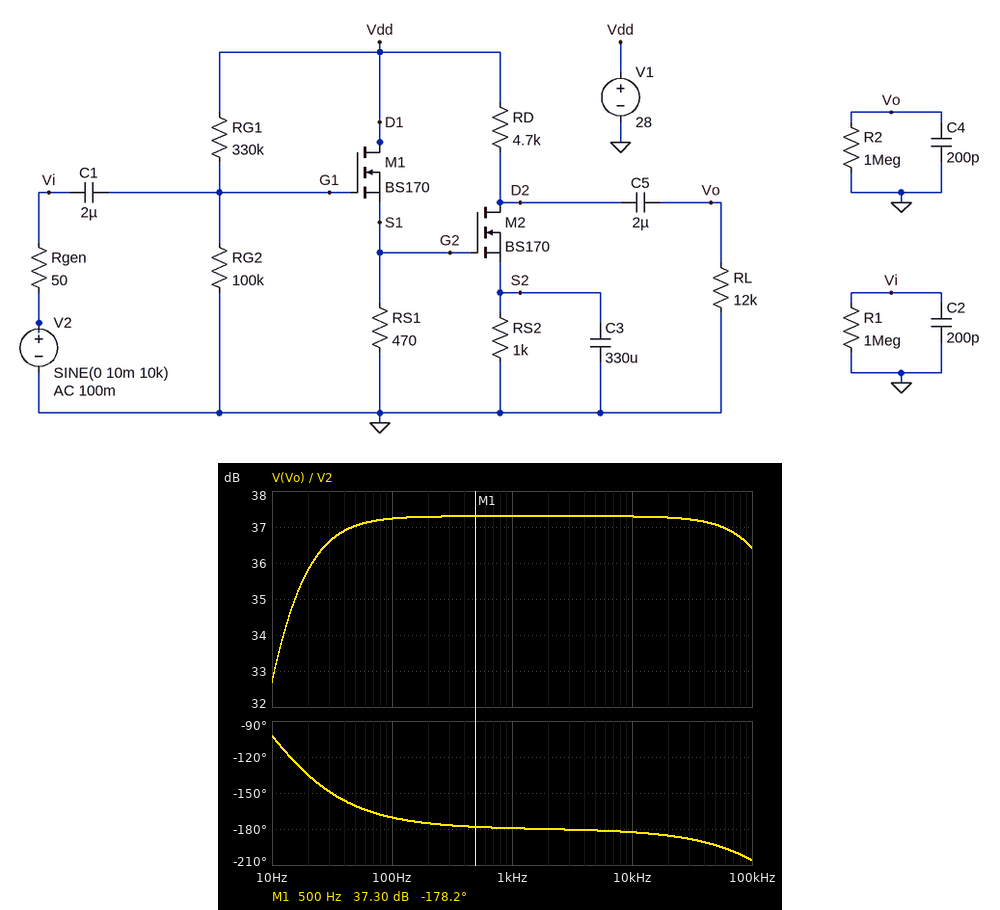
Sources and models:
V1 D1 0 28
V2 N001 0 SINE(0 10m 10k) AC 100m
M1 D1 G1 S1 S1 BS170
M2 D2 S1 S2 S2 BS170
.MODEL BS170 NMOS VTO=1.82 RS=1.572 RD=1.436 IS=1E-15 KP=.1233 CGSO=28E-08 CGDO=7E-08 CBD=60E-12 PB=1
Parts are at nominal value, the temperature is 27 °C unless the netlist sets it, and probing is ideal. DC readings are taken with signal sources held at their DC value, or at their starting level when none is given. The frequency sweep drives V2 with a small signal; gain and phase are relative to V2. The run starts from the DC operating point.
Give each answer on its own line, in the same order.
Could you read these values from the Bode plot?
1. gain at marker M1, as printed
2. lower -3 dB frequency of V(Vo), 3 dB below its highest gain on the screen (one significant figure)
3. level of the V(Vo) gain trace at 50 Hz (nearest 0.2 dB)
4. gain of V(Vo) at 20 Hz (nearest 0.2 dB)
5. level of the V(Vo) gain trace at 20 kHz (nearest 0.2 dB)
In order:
37.30 dB
10 Hz
37.0 dB
35.8 dB
37.2 dB
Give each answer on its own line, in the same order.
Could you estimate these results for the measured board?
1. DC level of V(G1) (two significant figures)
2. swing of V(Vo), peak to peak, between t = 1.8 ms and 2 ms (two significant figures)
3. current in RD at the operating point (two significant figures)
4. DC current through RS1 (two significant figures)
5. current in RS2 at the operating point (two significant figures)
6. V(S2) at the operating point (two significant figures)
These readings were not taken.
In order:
6.5 V
1.5 V
2.3 mA
9.1 mA
2.3 mA
2.3 V
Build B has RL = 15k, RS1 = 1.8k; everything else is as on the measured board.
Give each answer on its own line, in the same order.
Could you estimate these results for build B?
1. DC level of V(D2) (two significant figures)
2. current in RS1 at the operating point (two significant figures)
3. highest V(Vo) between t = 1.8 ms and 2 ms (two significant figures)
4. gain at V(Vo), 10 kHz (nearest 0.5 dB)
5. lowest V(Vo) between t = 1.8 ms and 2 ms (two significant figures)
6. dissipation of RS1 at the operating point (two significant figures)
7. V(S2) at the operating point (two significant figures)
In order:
16 V
2.5 mA
810 mV
38.5 dB
-840 mV
11 mW
2.5 V
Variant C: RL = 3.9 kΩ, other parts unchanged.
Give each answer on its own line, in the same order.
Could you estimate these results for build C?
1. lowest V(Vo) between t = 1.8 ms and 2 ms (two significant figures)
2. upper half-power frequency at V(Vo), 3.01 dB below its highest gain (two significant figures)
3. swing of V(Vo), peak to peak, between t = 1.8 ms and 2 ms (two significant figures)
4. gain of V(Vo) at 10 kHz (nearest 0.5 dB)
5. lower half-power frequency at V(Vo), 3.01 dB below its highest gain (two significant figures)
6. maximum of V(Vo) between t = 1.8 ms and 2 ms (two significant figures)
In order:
-470 mV
330 kHz
930 mV
33.5 dB
16 Hz
450 mV
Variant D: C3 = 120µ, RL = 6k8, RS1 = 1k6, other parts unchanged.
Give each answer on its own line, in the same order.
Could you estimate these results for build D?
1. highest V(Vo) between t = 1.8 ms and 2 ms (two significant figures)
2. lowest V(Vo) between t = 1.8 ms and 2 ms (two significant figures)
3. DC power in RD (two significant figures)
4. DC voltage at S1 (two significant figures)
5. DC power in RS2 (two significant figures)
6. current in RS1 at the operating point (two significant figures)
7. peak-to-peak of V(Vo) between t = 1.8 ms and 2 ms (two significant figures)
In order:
630 mV
-650 mV
28 mW
4.5 V
6.0 mW
2.8 mA
1.3 V
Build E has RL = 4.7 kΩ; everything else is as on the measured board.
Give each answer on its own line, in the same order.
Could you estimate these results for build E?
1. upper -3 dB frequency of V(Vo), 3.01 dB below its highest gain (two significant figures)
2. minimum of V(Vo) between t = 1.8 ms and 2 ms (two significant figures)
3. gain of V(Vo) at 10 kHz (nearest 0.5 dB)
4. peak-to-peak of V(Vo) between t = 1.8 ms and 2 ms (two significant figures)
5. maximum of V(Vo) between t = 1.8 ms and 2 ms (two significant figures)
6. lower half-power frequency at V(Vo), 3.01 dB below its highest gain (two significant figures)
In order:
300 kHz
-520 mV
34.0 dB
1.0 V
500 mV
16 Hz
